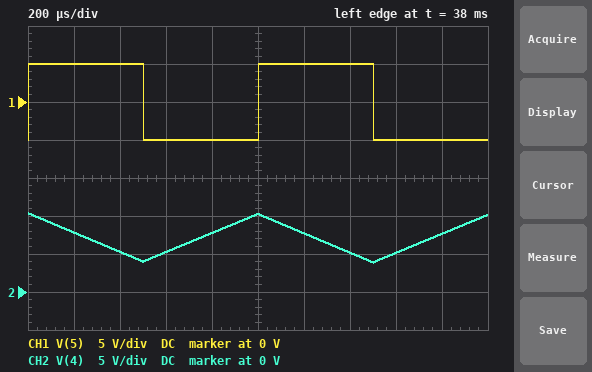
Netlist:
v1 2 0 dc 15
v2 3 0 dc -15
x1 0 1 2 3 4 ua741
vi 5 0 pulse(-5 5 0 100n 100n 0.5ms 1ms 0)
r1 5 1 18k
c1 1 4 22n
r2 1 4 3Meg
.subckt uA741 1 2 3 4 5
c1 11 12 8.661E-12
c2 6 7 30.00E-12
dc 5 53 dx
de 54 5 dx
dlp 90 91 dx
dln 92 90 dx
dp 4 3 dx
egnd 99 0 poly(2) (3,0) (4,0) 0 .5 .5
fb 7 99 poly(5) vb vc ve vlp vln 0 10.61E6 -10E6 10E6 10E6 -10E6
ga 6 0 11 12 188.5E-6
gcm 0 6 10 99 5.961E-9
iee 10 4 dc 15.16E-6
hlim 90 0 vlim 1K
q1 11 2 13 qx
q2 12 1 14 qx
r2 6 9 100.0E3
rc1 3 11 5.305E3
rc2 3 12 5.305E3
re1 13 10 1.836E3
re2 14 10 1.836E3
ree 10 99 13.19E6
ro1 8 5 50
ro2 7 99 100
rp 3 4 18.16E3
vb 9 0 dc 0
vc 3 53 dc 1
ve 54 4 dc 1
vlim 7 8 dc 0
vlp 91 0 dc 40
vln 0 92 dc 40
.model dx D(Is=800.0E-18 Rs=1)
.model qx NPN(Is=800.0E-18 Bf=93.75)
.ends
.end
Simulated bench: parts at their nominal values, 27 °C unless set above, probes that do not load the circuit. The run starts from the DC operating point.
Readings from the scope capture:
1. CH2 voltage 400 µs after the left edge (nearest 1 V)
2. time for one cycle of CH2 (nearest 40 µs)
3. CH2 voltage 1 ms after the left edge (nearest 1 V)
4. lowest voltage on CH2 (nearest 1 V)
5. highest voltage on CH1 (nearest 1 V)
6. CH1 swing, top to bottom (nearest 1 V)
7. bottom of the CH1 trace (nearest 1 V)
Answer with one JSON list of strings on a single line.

["5 V", "1.00 ms", "10 V", "4 V", "5 V", "10 V", "-5 V"]
